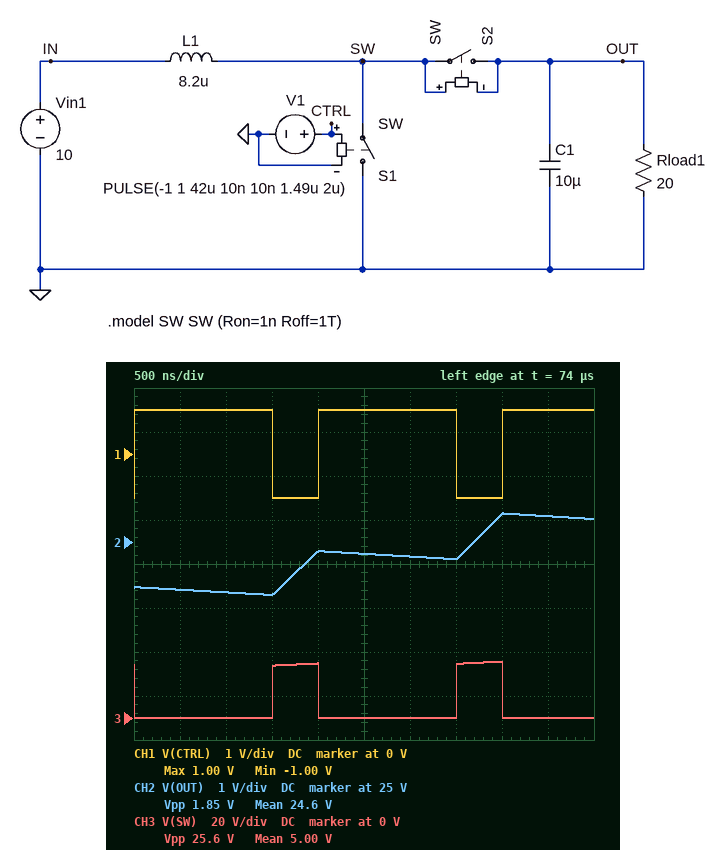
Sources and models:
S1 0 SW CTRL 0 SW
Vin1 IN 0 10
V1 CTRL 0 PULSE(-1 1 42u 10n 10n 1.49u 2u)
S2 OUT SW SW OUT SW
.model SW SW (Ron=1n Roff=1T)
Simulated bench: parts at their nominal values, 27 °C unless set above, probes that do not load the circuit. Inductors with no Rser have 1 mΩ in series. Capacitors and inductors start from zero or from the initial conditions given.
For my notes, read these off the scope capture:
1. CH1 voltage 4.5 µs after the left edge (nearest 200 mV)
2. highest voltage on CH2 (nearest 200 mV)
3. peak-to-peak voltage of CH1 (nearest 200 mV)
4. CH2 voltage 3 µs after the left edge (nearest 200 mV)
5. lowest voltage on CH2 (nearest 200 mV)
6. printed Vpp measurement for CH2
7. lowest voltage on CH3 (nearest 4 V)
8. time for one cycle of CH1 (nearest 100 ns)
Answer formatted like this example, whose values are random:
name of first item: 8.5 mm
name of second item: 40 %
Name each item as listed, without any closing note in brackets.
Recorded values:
CH1 voltage 4.5 µs after the left edge: 1.0 V
highest voltage on CH2: 25.6 V
peak-to-peak voltage of CH1: 2.0 V
CH2 voltage 3 µs after the left edge: 24.6 V
lowest voltage on CH2: 23.8 V
printed Vpp measurement for CH2: 1.85 V
lowest voltage on CH3: 0 V
time for one cycle of CH1: 2.0 µs
